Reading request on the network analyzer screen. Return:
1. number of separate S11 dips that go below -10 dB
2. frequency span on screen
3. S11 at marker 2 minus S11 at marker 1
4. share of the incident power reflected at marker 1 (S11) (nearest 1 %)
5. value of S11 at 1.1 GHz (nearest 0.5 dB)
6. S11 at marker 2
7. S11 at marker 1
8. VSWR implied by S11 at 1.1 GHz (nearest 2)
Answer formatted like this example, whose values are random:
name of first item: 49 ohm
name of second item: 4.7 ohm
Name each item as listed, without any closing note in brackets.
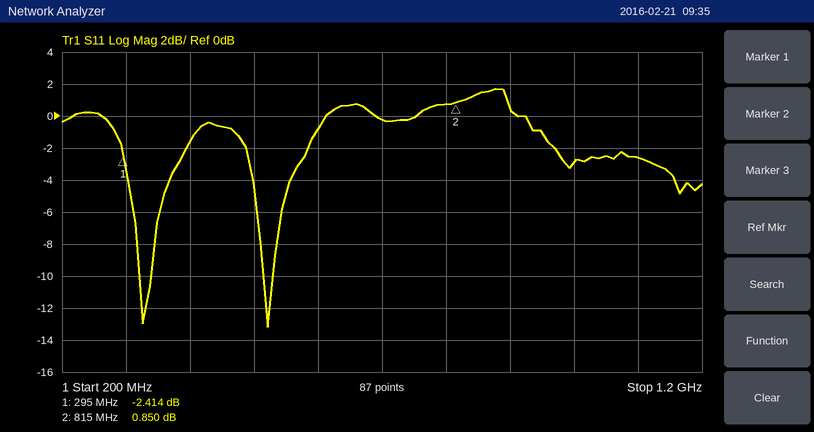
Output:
number of separate S11 dips that go below -10 dB: 2
frequency span on screen: 1 GHz
S11 at marker 2 minus S11 at marker 1: 3.264 dB
share of the incident power reflected at marker 1 (S11): 57 %
value of S11 at 1.1 GHz: -2.5 dB
S11 at marker 2: 0.850 dB
S11 at marker 1: -2.414 dB
VSWR implied by S11 at 1.1 GHz: 6
